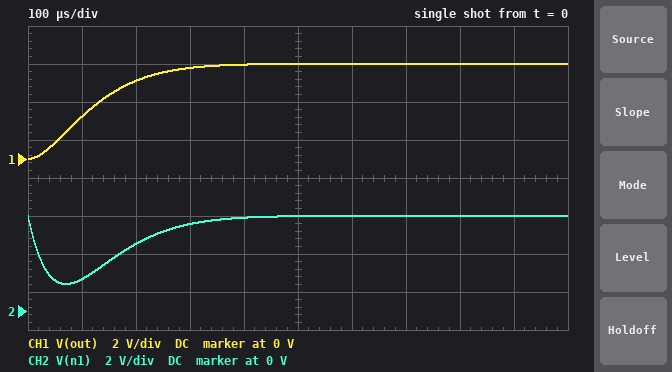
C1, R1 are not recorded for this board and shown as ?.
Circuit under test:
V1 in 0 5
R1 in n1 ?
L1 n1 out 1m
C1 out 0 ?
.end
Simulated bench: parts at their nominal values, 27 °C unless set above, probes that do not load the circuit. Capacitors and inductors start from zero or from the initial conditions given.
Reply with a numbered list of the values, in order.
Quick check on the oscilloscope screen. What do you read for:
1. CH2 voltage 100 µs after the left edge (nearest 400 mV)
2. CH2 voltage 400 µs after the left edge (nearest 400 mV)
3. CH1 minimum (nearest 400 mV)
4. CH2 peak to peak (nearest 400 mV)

1. 1.6 V
2. 4.8 V
3. 0 V
4. 3.6 V
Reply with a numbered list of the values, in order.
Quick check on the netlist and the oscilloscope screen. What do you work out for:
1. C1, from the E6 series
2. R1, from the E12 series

1. 4.7 µF
2. 27 Ω
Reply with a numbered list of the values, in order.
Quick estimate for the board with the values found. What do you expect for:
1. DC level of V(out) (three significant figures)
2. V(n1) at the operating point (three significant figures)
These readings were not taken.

1. 5.00 V
2. 5.00 V
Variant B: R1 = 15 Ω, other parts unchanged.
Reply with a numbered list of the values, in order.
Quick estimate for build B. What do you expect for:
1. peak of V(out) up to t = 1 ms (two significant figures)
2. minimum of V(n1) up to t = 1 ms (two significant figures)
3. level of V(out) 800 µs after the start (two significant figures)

1. 5.8 V
2. 2.2 V
3. 5.0 V
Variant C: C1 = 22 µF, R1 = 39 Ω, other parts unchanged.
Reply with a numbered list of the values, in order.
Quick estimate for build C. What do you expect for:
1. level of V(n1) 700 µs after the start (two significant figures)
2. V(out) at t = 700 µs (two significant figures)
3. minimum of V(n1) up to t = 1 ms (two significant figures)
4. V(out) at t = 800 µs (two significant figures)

1. 2.7 V
2. 2.8 V
3. 390 mV
4. 3.0 V
